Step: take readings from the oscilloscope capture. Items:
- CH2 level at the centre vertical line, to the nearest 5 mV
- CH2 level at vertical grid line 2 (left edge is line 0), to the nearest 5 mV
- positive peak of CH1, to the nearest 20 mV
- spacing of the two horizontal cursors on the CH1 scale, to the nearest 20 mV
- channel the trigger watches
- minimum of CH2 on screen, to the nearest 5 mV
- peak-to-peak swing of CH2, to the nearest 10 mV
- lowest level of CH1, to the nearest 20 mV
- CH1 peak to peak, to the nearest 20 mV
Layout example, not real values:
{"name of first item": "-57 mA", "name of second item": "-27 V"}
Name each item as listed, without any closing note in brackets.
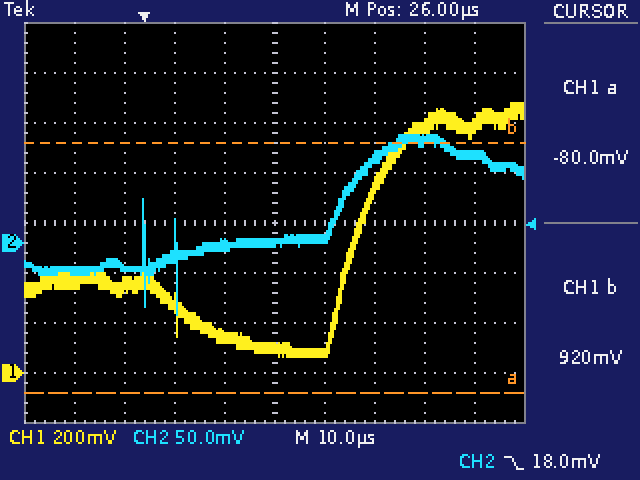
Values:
{"CH2 level at the centre vertical line, to the nearest 5 mV": "0 mV", "CH2 level at vertical grid line 2 (left edge is line 0), to the nearest 5 mV": "-25 mV", "positive peak of CH1, to the nearest 20 mV": "1.08 V", "spacing of the two horizontal cursors on the CH1 scale, to the nearest 20 mV": "1.00 V", "channel the trigger watches": "CH2", "minimum of CH2 on screen, to the nearest 5 mV": "-70 mV", "peak-to-peak swing of CH2, to the nearest 10 mV": "180 mV", "lowest level of CH1, to the nearest 20 mV": "60 mV", "CH1 peak to peak, to the nearest 20 mV": "1.02 V"}
